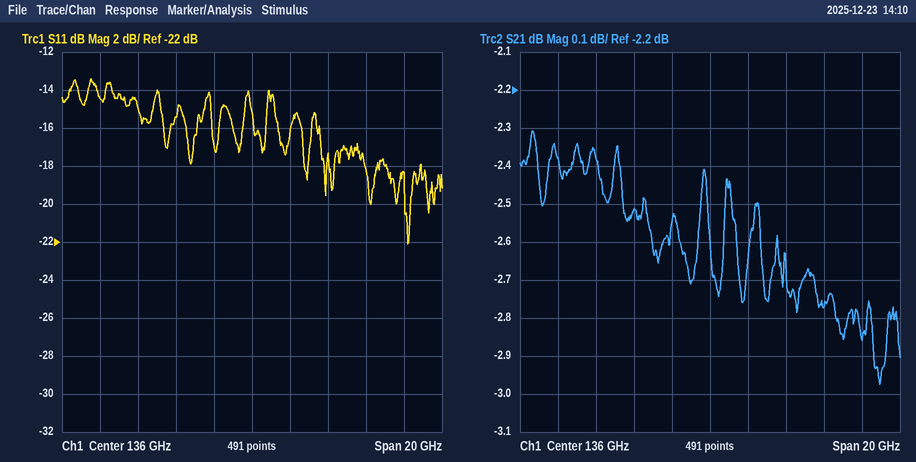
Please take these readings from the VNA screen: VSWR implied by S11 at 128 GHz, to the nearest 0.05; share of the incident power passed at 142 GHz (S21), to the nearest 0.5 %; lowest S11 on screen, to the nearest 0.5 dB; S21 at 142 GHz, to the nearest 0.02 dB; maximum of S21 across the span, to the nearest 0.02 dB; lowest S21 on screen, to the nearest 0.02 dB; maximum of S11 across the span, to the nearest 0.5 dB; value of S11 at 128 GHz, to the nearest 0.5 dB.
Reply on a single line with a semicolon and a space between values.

1.45; 53.0 %; -22.0 dB; -2.76 dB; -2.30 dB; -2.98 dB; -13.5 dB; -14.5 dB
